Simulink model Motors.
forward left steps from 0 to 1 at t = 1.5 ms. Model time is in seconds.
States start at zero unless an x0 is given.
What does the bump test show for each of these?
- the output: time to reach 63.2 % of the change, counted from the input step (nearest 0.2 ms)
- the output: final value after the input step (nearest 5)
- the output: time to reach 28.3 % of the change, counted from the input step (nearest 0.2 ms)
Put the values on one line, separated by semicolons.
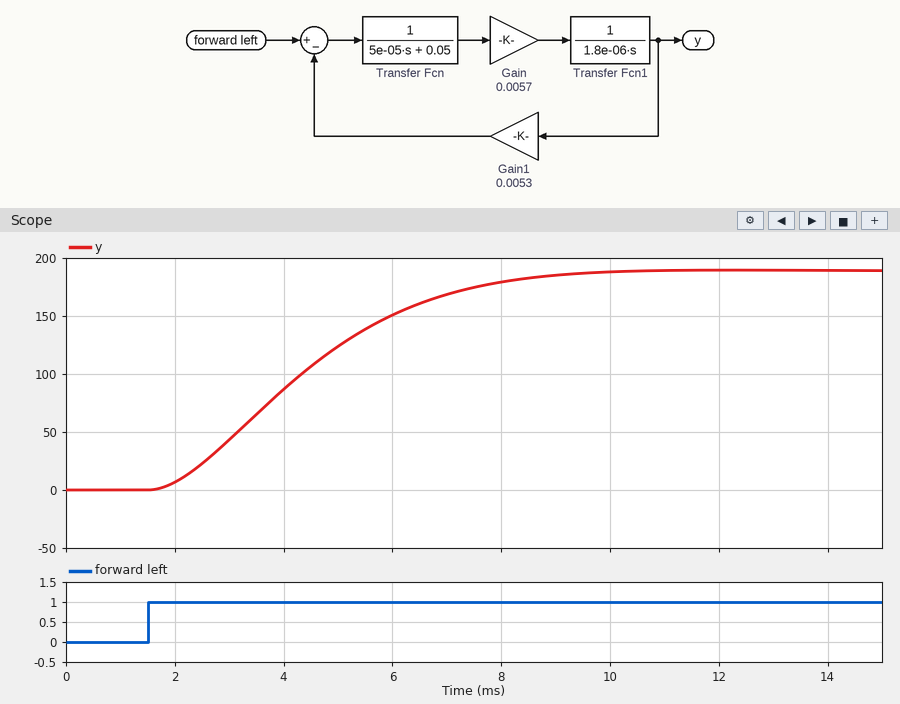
3.4 ms; 190; 1.8 ms
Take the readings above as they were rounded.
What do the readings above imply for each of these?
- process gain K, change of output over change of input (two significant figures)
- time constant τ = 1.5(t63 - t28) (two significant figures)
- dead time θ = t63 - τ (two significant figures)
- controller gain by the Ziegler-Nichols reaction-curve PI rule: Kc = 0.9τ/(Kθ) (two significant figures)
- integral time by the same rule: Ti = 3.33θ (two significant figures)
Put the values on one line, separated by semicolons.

190; 2.4 ms; 1.0 ms; 0.011; 3.3 ms
